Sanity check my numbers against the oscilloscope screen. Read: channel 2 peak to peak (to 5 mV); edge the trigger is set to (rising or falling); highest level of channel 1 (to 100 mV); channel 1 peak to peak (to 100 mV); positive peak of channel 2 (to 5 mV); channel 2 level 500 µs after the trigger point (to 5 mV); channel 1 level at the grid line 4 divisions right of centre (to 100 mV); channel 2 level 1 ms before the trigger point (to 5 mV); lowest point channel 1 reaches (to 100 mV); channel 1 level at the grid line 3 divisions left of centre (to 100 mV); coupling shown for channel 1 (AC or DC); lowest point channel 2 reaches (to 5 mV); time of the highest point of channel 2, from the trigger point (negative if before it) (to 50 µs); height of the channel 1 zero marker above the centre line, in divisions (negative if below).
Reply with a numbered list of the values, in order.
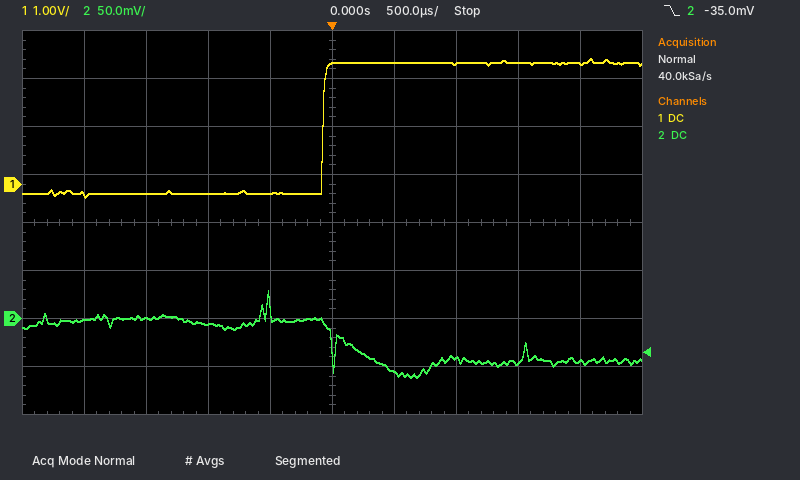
1. 90 mV
2. falling
3. 2.6 V
4. 2.9 V
5. 30 mV
6. -55 mV
7. 2.5 V
8. -5 mV
9. -300 mV
10. -200 mV
11. DC
12. -60 mV
13. -500 µs
14. +0.8 div
